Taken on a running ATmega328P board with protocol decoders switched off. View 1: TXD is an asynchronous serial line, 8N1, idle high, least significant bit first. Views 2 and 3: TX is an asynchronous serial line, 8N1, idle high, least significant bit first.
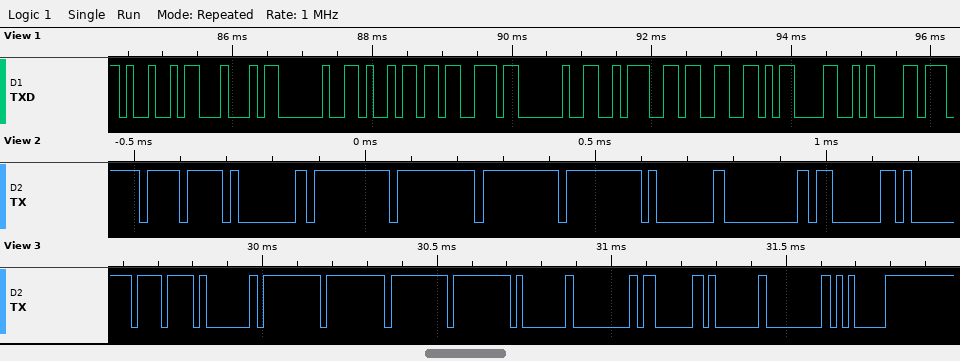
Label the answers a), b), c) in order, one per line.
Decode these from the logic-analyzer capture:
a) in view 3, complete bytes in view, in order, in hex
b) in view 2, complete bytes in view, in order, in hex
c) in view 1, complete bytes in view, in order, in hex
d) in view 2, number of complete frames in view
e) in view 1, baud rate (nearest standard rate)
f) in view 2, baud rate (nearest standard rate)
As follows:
a) 0xEF 0x01 0xFF 0xFF 0xFF 0xFF 0x01 0x00 0x03 0x01 0x00 0x05
b) EF 01 FF FF FF FF 01 00 03
c) 0x49 0x44 0x20 0x69 0x73 0x20 0x3A 0x33 0x0D 0x0A
d) 9
e) 9600 baud
f) 57600 baud
